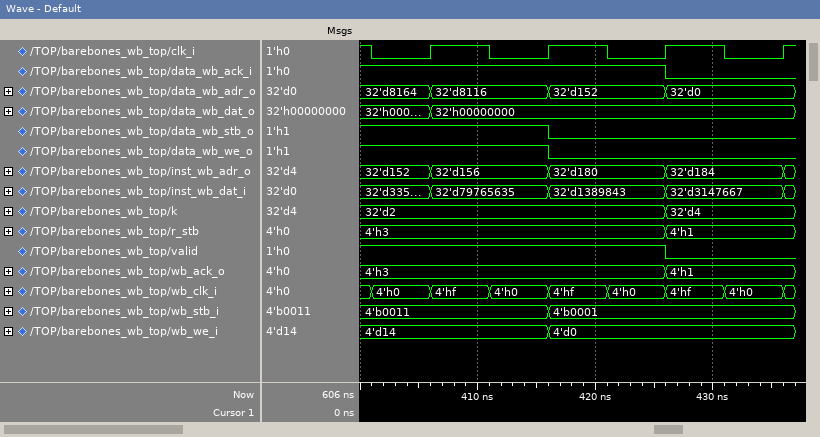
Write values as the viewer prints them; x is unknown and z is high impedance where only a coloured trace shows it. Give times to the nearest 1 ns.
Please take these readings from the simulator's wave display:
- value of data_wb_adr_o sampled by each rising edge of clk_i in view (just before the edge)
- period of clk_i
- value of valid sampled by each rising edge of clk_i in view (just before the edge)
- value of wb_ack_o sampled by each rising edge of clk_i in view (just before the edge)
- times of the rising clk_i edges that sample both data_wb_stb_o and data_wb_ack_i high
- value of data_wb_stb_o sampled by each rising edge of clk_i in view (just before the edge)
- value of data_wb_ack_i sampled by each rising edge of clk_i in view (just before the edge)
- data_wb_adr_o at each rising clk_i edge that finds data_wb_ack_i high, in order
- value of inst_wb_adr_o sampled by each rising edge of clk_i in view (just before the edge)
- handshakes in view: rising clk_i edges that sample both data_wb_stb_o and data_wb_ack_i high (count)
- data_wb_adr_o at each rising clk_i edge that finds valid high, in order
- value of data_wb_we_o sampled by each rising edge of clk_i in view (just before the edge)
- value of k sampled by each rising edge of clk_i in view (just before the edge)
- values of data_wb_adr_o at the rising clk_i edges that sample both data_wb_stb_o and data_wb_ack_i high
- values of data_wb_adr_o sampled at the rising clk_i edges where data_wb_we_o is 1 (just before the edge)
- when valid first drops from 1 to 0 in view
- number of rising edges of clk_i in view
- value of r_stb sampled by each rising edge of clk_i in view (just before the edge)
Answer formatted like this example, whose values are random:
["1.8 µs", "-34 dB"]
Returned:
["32'd8164, 32'd8116, 32'd152, 32'd0", "10 ns", "1 1 1 0", "4'h3, 4'h3, 4'h3, 4'h1", "406 ns, 416 ns", "1 1 0 0", "1 1 1 0", "32'd8164, 32'd8116, 32'd152", "32'd152, 32'd156, 32'd180, 32'd184", "2", "32'd8164, 32'd8116, 32'd152", "1 1 0 0", "32'd2, 32'd2, 32'd2, 32'd4", "32'd8164, 32'd8116", "32'd8164, 32'd8116", "426 ns", "4", "4'h3, 4'h3, 4'h3, 4'h1"]
